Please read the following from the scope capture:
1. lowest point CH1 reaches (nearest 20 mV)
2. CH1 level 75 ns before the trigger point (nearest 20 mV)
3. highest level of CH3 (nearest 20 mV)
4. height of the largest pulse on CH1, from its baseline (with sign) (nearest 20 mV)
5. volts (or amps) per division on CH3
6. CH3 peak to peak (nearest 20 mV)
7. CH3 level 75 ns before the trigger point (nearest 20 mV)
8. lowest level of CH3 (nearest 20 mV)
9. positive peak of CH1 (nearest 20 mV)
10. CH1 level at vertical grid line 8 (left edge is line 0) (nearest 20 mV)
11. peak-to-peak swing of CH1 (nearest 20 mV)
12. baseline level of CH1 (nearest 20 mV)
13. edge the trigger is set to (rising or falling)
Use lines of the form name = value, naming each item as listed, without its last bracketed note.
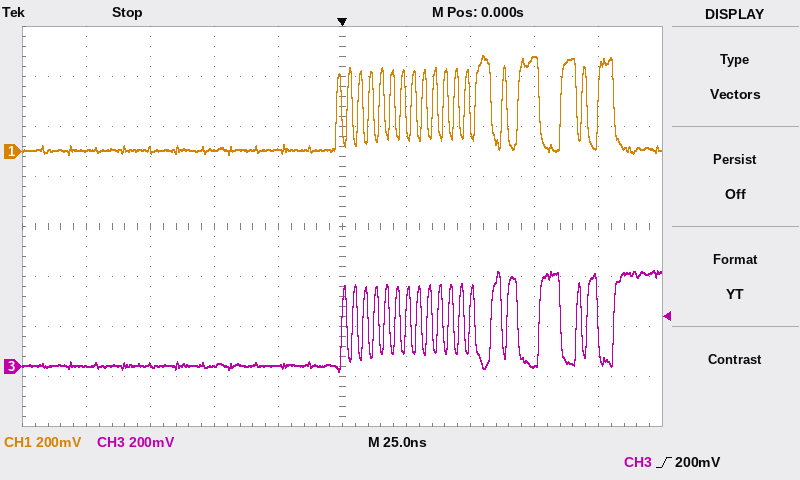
lowest point CH1 reaches = -20 mV
CH1 level 75 ns before the trigger point = 0 mV
highest level of CH3 = 380 mV
height of the largest pulse on CH1, from its baseline (with sign) = +380 mV
volts (or amps) per division on CH3 = 200 mV
CH3 peak to peak = 400 mV
CH3 level 75 ns before the trigger point = 0 mV
lowest level of CH3 = -20 mV
positive peak of CH1 = 380 mV
CH1 level at vertical grid line 8 (left edge is line 0) = 380 mV
peak-to-peak swing of CH1 = 400 mV
baseline level of CH1 = 0 mV
edge the trigger is set to = rising
